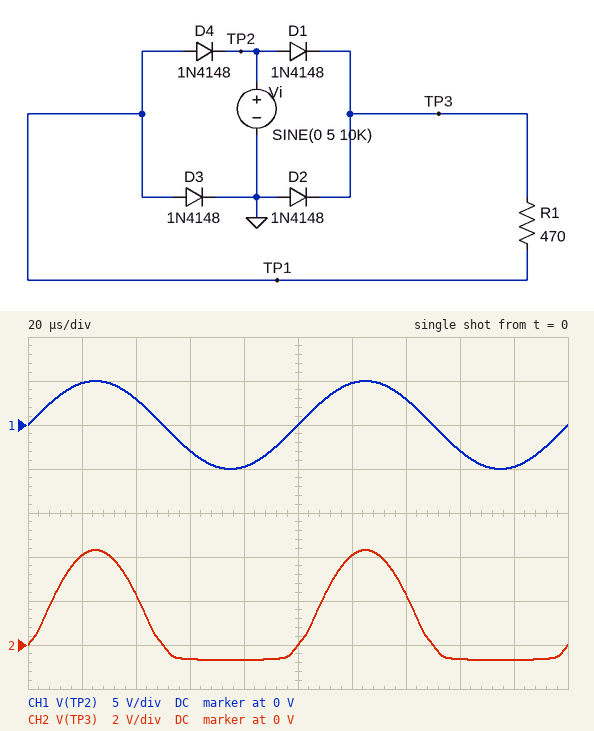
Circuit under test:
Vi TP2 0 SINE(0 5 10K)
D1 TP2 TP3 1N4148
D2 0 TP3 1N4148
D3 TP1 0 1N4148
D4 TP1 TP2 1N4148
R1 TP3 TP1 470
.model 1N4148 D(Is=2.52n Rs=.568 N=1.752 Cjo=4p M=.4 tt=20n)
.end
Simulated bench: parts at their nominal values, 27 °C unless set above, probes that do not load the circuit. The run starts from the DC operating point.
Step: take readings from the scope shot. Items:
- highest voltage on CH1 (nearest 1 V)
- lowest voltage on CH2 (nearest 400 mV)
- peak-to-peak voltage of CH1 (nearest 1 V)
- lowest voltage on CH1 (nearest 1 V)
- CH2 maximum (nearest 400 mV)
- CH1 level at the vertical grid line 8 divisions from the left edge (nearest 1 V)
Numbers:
5 V
-800 mV
10 V
-5 V
4.4 V
-3 V
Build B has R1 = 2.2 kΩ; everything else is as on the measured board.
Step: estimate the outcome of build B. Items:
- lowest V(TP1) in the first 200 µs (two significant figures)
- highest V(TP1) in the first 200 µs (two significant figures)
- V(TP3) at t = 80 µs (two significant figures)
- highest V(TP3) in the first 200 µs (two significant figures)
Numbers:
-4.4 V
610 mV
-610 mV
4.4 V
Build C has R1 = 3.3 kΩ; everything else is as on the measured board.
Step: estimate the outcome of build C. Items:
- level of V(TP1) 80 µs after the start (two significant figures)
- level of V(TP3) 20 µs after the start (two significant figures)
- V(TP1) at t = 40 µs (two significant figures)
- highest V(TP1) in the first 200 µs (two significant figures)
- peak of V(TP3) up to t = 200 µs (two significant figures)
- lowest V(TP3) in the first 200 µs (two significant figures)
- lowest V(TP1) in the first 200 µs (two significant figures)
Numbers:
-4.2 V
4.2 V
560 mV
590 mV
4.4 V
-590 mV
-4.4 V
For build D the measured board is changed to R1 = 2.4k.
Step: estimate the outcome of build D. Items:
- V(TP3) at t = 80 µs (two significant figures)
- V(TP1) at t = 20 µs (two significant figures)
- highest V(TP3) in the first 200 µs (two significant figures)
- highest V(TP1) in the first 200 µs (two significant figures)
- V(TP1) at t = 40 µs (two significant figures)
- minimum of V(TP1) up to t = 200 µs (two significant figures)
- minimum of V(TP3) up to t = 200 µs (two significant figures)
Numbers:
-600 mV
600 mV
4.4 V
610 mV
570 mV
-4.4 V
-610 mV
